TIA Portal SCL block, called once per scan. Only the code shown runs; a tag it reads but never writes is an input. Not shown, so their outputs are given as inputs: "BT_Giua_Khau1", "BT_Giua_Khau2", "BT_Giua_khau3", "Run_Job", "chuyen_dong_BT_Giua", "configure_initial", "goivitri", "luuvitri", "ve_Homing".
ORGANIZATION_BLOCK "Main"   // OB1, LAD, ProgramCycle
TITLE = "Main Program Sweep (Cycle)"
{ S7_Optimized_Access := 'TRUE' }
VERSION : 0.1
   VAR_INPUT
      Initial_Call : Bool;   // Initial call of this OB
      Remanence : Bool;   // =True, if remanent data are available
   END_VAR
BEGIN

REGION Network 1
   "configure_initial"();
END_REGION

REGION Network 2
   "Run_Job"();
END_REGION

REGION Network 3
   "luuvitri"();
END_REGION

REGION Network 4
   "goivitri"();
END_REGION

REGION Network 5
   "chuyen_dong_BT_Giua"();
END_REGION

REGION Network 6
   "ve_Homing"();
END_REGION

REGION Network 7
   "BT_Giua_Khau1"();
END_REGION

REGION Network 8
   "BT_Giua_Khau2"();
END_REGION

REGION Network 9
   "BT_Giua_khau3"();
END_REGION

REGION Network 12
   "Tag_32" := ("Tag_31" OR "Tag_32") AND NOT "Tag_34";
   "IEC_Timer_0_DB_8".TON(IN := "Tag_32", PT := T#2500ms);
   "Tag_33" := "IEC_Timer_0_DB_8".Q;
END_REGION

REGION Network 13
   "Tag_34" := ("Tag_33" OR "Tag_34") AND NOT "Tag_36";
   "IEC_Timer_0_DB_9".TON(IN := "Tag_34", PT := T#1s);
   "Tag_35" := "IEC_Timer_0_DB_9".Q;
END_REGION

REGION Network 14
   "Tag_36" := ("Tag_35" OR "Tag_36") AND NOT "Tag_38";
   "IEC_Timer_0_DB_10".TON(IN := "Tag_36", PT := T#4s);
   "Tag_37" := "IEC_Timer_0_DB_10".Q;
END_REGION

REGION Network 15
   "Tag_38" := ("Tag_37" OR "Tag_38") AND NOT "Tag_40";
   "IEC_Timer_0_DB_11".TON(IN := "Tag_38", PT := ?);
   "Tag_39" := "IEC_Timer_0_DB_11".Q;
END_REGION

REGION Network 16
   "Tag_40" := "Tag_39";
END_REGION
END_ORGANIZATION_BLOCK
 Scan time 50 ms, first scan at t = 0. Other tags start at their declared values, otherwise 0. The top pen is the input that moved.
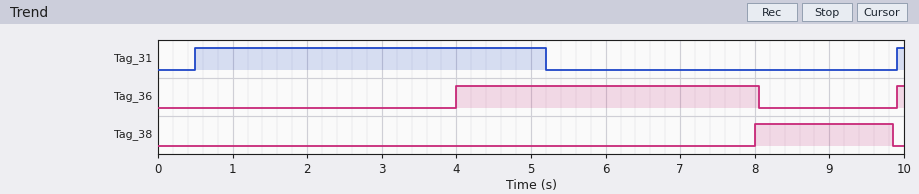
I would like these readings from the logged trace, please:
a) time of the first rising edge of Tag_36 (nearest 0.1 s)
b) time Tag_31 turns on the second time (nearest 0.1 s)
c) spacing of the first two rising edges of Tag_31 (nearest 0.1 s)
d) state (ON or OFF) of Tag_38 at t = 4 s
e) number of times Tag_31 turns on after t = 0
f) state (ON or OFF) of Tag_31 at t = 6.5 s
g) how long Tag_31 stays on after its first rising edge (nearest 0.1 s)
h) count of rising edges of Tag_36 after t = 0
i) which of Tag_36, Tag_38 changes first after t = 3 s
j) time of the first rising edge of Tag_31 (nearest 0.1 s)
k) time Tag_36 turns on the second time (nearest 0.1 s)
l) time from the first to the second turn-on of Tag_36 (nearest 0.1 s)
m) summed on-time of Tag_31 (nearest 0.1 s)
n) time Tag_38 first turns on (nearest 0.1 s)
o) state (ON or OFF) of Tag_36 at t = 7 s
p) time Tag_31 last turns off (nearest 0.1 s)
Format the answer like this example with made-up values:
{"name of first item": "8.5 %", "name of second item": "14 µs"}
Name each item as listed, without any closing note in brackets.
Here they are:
{"time of the first rising edge of Tag_36": "4.0 s", "time Tag_31 turns on the second time": "9.9 s", "spacing of the first two rising edges of Tag_31": "9.4 s", "state (ON or OFF) of Tag_38 at t = 4 s": "OFF", "number of times Tag_31 turns on after t = 0": "2", "state (ON or OFF) of Tag_31 at t = 6.5 s": "OFF", "how long Tag_31 stays on after its first rising edge": "4.7 s", "count of rising edges of Tag_36 after t = 0": "2", "which of Tag_36, Tag_38 changes first after t = 3 s": "Tag_36", "time of the first rising edge of Tag_31": "0.5 s", "time Tag_36 turns on the second time": "9.9 s", "time from the first to the second turn-on of Tag_36": "5.9 s", "summed on-time of Tag_31": "4.8 s", "time Tag_38 first turns on": "8.0 s", "state (ON or OFF) of Tag_36 at t = 7 s": "ON", "time Tag_31 last turns off": "5.2 s"}
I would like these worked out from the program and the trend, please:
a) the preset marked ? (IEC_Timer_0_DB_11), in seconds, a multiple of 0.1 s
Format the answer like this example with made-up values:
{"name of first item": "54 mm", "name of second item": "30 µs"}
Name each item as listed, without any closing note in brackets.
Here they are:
{"the preset marked ? (IEC_Timer_0_DB_11), in seconds, a multiple of 0.1 s": "1.8 s"}
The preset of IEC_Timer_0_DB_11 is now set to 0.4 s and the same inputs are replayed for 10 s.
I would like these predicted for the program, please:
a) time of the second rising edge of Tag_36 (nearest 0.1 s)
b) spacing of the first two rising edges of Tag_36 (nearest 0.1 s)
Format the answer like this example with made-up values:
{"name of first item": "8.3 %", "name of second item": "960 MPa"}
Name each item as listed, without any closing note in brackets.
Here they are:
{"time of the second rising edge of Tag_36": "9.1 s", "spacing of the first two rising edges of Tag_36": "5.1 s"}
